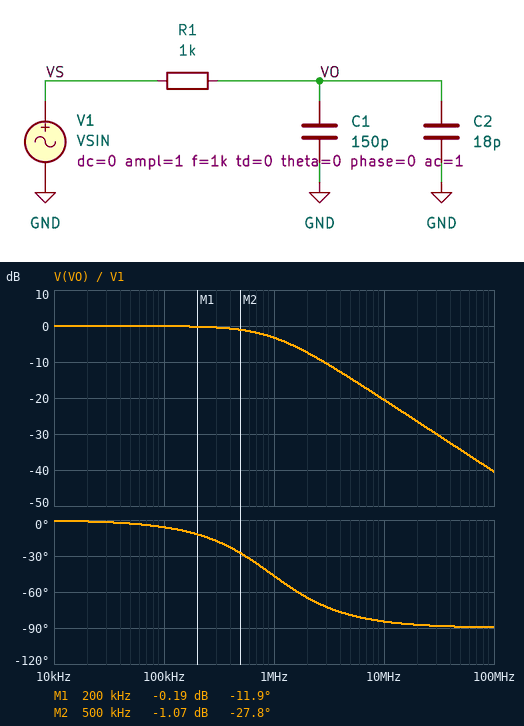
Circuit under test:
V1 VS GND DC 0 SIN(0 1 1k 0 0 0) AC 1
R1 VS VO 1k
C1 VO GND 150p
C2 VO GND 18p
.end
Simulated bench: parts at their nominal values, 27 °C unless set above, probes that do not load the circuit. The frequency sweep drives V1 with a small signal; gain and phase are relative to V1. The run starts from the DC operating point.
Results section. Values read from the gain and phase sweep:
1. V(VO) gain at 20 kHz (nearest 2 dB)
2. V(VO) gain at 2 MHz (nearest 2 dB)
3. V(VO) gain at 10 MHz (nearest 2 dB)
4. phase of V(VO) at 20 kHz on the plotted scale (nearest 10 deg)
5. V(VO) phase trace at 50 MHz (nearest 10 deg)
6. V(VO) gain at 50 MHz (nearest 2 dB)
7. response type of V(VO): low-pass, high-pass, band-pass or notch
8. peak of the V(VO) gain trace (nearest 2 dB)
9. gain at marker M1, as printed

0 dB
-8 dB
-20 dB
0 deg
-90 deg
-34 dB
low-pass
0 dB
-0.19 dB
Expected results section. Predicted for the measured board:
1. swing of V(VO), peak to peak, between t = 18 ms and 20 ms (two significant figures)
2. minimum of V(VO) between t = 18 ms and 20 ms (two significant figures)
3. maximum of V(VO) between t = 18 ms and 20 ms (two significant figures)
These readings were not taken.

2.0 V
-1.0 V
1.0 V
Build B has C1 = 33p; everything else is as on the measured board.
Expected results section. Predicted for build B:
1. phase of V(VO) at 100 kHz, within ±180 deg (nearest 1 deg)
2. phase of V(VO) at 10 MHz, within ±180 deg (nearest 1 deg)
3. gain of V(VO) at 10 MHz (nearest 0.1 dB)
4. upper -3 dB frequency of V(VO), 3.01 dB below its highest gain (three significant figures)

-2 deg
-73 deg
-10.5 dB
3.12 MHz
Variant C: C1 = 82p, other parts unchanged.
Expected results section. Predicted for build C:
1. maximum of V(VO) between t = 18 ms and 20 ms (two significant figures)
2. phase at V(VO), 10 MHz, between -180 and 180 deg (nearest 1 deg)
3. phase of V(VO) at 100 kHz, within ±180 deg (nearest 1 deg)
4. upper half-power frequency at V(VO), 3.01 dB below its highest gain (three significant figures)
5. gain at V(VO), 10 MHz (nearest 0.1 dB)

1.0 V
-81 deg
-4 deg
1.59 MHz
-16.1 dB
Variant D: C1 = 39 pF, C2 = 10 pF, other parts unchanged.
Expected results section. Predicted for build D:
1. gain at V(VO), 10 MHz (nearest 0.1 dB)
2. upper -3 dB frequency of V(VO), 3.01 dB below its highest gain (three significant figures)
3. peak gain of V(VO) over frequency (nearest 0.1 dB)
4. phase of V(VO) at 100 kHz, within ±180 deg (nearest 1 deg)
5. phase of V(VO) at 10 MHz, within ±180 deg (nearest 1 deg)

-10.2 dB
3.25 MHz
0 dB
-2 deg
-72 deg
